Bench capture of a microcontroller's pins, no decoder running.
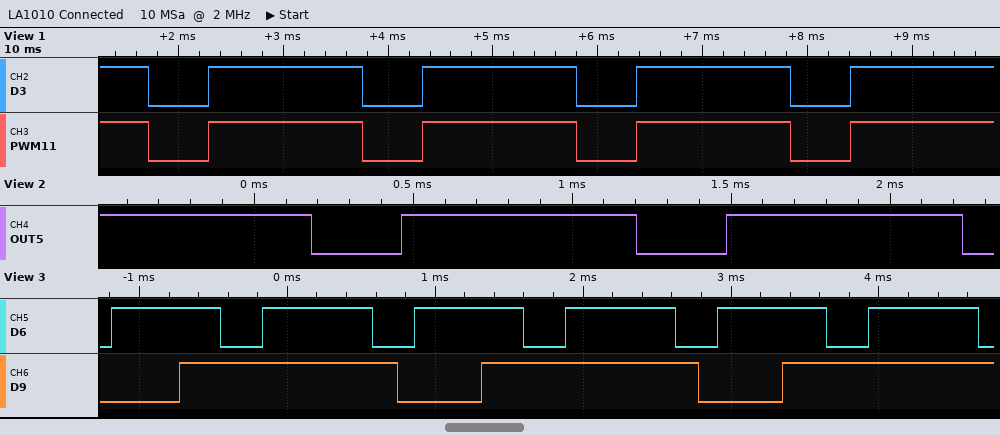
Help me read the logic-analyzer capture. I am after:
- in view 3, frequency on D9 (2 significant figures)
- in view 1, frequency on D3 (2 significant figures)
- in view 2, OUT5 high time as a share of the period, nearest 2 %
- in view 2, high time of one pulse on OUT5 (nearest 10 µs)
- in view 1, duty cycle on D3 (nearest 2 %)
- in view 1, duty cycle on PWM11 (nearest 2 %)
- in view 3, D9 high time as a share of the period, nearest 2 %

490 Hz
490 Hz
72 %
740 µs
72 %
72 %
72 %
